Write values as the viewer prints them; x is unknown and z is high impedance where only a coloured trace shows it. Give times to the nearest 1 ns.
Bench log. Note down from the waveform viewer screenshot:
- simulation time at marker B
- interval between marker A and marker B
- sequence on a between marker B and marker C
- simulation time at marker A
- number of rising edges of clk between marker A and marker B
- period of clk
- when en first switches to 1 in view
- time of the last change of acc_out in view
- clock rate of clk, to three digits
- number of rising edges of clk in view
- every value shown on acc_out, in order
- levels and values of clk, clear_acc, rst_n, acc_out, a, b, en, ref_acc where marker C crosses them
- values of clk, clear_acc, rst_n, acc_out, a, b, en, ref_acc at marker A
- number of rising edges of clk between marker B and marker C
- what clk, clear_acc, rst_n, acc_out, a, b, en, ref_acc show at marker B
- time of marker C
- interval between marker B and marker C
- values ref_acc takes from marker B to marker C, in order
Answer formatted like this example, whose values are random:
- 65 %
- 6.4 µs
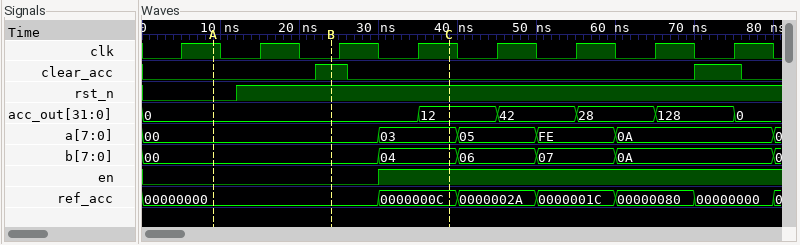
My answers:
- 24 ns
- 15 ns
- 00, 03
- 9 ns
- 1
- 10 ns
- 30 ns
- 75 ns
- 100 MHz
- 8
- 0, 12, 42, 28, 128, 0
- clk=1, clear_acc=0, rst_n=1, acc_out=12, a=03, b=04, en=1, ref_acc=0000000C
- clk=1, clear_acc=0, rst_n=0, acc_out=0, a=00, b=00, en=0, ref_acc=00000000
- 2
- clk=0, clear_acc=1, rst_n=1, acc_out=0, a=00, b=00, en=0, ref_acc=00000000
- 39 ns
- 15 ns
- 00000000, 0000000C
